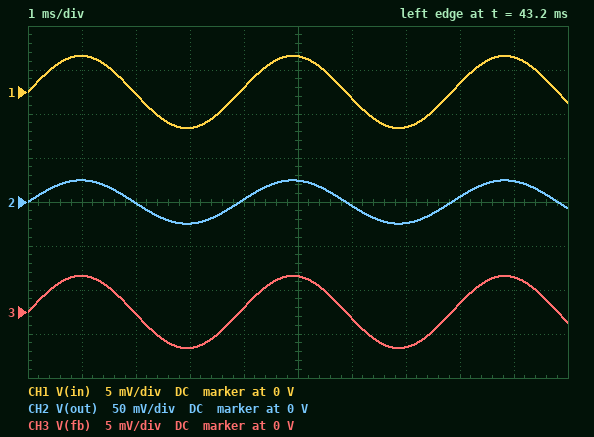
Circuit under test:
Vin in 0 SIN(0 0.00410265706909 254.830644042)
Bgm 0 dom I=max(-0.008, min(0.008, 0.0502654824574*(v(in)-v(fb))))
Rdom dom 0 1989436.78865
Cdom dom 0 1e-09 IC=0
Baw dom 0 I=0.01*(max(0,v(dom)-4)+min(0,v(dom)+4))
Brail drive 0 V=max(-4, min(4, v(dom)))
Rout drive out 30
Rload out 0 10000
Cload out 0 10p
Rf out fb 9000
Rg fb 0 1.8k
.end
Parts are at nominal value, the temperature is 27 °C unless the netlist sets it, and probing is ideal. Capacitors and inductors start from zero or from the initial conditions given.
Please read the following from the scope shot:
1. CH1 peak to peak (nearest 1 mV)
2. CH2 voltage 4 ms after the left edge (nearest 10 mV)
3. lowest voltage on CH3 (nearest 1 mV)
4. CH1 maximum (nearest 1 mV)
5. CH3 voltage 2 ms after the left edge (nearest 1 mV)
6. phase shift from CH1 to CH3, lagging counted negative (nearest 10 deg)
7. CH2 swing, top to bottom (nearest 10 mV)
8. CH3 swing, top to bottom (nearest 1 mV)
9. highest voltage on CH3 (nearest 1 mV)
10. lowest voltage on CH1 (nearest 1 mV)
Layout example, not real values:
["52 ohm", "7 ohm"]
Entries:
["8 mV", "0 V", "-4 mV", "4 mV", "0 V", "0 deg", "50 mV", "8 mV", "4 mV", "-4 mV"]
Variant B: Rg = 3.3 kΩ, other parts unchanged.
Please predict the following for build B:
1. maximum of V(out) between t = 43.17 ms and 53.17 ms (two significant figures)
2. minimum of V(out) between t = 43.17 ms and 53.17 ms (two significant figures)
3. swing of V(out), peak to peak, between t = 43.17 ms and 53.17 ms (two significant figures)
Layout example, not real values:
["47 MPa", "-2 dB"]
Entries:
["15 mV", "-15 mV", "31 mV"]
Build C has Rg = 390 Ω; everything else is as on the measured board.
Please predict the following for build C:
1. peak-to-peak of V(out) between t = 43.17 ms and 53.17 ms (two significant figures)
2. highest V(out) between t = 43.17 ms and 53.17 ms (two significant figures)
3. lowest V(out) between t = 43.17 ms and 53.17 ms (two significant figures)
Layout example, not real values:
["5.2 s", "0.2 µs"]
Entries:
["200 mV", "99 mV", "-99 mV"]
